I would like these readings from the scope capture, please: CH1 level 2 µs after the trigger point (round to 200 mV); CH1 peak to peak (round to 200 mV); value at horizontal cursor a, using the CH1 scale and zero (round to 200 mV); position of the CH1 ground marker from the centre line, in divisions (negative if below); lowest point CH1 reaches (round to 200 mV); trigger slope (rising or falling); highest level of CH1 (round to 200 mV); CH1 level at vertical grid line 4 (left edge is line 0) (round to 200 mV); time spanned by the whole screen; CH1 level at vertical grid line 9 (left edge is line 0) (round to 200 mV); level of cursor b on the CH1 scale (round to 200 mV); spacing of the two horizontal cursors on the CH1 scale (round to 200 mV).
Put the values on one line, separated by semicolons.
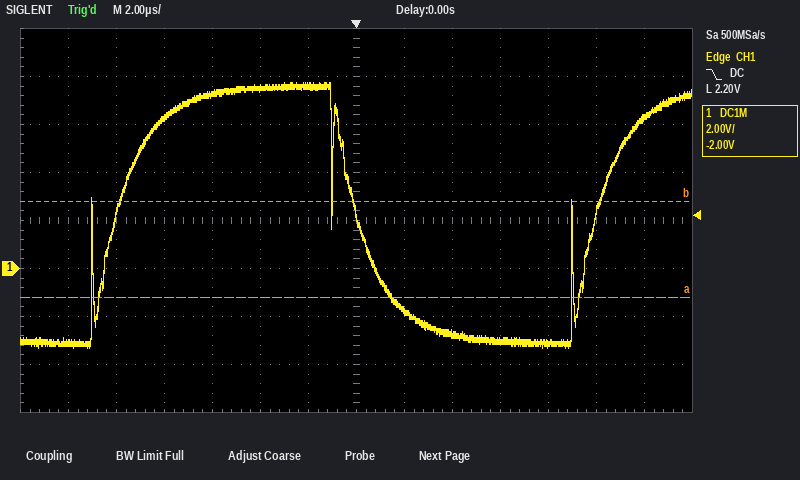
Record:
-1.8 V; 11.0 V; -1.2 V; -1.0 div; -3.2 V; falling; 7.8 V; 7.2 V; 28 µs; -2.8 V; 2.8 V; 4.0 V
